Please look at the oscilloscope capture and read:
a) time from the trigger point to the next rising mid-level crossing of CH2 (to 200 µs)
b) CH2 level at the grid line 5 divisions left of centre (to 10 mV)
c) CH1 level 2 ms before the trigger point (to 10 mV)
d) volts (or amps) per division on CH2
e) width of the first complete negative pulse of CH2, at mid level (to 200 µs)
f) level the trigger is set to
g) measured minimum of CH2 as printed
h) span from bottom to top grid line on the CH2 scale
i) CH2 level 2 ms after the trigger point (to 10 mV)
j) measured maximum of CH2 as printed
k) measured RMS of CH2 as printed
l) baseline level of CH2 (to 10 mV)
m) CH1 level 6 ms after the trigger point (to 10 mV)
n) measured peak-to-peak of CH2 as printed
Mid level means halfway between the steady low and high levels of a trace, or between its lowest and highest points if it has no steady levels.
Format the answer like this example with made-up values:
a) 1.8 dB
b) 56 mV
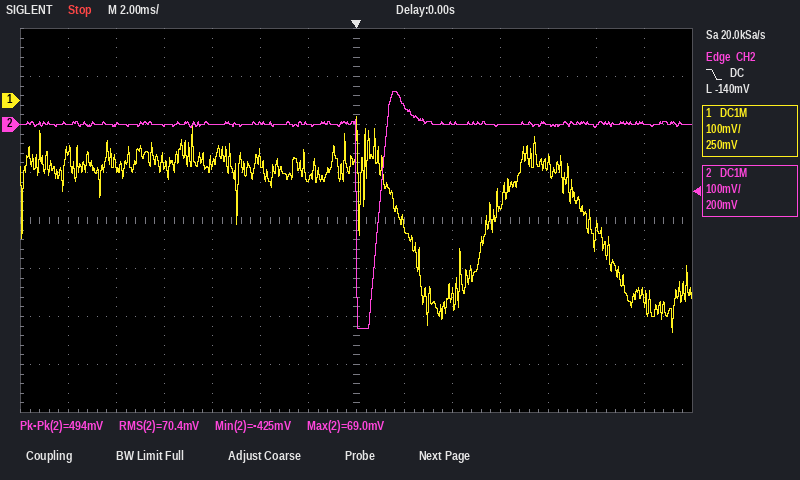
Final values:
a) 1.0 ms
b) 0 mV
c) -160 mV
d) 100 mV
e) 1.0 ms
f) -140 mV
g) -425 mV
h) 800 mV
i) 40 mV
j) 69.0 mV
k) 70.4 mV
l) 0 mV
m) -220 mV
n) 494 mV
